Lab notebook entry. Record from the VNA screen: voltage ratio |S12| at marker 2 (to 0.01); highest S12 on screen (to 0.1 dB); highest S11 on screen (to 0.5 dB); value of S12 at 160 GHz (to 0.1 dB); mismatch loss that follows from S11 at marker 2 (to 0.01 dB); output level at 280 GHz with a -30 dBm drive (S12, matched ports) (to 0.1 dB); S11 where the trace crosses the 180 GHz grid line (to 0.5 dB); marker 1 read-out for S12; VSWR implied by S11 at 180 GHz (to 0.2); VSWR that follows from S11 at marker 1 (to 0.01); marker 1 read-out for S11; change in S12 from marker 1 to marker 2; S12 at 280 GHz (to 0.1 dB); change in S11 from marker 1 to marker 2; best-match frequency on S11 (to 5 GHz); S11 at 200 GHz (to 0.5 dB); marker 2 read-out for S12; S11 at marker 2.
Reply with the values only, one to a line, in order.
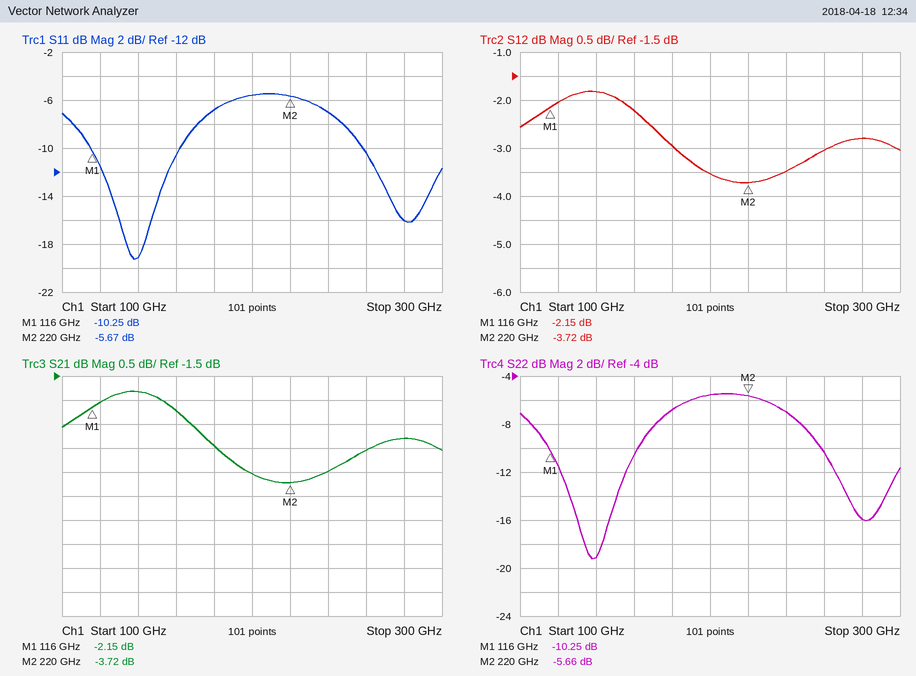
0.65
-1.8 dB
-5.5 dB
-2.2 dB
1.37 dB
-32.8 dBm
-7.0 dB
-2.15 dB
2.6
1.89
-10.25 dB
-1.57 dB
-2.8 dB
4.58 dB
140 GHz
-5.5 dB
-3.72 dB
-5.67 dB
